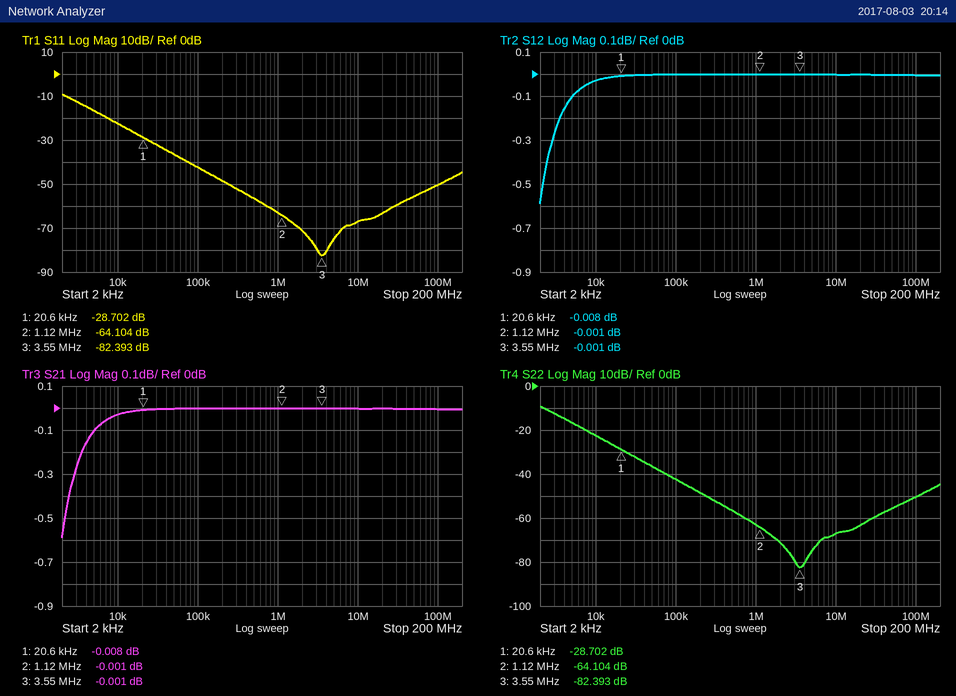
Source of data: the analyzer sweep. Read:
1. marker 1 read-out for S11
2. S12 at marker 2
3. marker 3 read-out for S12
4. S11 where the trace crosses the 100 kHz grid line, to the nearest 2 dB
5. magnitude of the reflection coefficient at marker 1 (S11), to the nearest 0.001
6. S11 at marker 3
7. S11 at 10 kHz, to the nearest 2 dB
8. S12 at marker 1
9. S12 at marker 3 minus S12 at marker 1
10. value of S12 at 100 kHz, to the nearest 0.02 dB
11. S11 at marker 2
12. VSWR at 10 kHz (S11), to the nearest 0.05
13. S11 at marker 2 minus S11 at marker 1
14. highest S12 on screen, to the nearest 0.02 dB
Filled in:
-28.702 dB
-0.001 dB
-0.001 dB
-42 dB
0.037
-82.393 dB
-22 dB
-0.008 dB
0.007 dB
0.00 dB
-64.104 dB
1.15
-35.402 dB
0.00 dB
